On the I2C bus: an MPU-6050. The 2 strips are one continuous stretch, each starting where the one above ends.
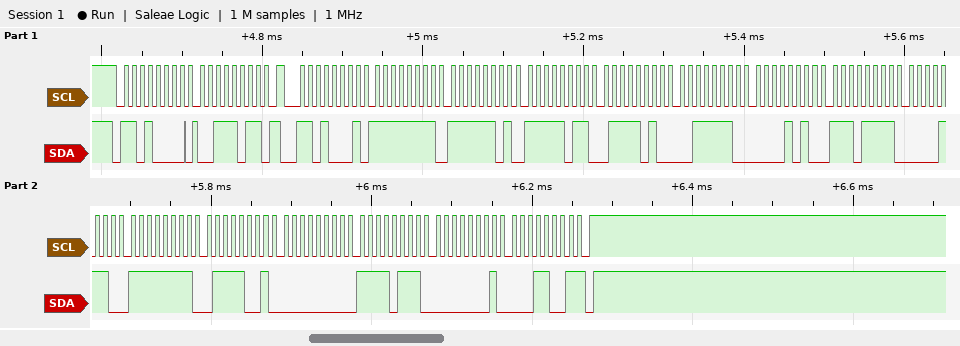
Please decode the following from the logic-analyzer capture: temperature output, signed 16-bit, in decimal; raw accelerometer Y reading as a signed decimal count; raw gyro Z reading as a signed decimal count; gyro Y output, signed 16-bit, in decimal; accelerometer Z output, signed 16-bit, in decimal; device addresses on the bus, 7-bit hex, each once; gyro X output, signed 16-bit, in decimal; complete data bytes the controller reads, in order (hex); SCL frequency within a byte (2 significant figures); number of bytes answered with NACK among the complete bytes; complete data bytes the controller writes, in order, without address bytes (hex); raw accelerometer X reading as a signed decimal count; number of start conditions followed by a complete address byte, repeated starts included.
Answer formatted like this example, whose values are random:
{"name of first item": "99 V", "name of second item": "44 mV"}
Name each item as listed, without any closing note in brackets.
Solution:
{"temperature output, signed 16-bit, in decimal": "-4338", "raw accelerometer Y reading as a signed decimal count": "-1158", "raw gyro Z reading as a signed decimal count": "281", "gyro Y output, signed 16-bit, in decimal": "247", "accelerometer Z output, signed 16-bit, in decimal": "15882", "device addresses on the bus, 7-bit hex, each once": "0x68", "gyro X output, signed 16-bit, in decimal": "-135", "complete data bytes the controller reads, in order": "FF FD FB 7A 3E 0A EF 0E FF 79 00 F7 01 19", "SCL frequency within a byte": "100 kHz", "number of bytes answered with NACK among the complete bytes": "1", "complete data bytes the controller writes, in order, without address bytes": "3B", "raw accelerometer X reading as a signed decimal count": "-3", "number of start conditions followed by a complete address byte, repeated starts included": "2"}
